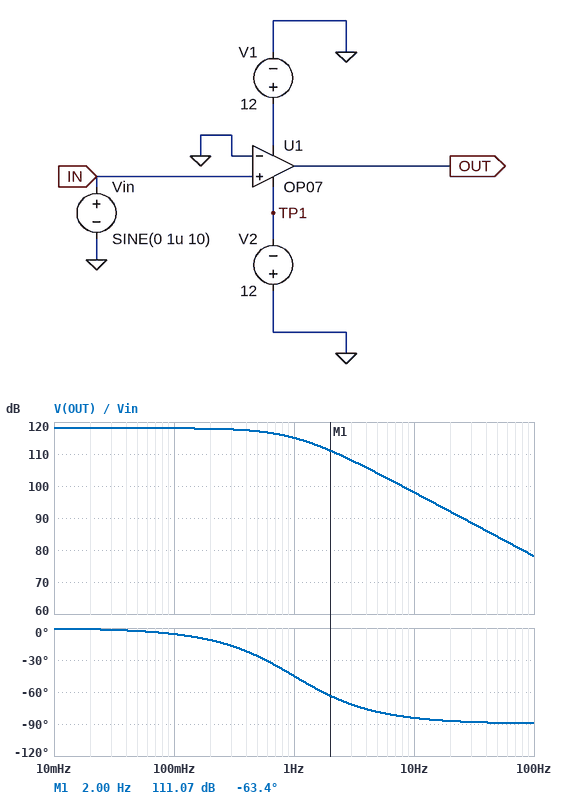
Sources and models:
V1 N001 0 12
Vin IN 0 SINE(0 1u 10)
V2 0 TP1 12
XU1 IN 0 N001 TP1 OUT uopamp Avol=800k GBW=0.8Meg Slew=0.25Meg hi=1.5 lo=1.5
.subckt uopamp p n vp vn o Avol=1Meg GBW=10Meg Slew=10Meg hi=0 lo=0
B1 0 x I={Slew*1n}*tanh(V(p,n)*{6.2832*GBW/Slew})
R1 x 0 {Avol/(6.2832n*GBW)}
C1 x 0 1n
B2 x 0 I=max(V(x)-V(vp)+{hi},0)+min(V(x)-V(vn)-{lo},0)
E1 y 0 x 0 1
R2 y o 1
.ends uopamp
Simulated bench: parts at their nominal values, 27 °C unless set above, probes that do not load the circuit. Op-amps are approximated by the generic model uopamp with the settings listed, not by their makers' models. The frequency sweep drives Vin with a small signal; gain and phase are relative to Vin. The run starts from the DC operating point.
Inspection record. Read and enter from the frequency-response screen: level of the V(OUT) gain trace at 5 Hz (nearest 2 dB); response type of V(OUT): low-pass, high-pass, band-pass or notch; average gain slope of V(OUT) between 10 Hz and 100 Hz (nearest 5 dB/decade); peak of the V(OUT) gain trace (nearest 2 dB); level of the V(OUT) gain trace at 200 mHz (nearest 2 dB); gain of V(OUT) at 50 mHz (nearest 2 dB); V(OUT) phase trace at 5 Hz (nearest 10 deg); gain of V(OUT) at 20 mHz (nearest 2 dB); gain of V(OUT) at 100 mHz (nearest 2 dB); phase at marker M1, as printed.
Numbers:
104 dB
low-pass
-20 dB/decade
118 dB
118 dB
118 dB
-80 deg
118 dB
118 dB
-63.4 deg
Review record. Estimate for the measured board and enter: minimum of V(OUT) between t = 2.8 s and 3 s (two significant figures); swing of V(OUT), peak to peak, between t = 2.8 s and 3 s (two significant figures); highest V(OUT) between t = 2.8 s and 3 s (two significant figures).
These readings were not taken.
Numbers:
-80 mV
160 mV
80 mV
